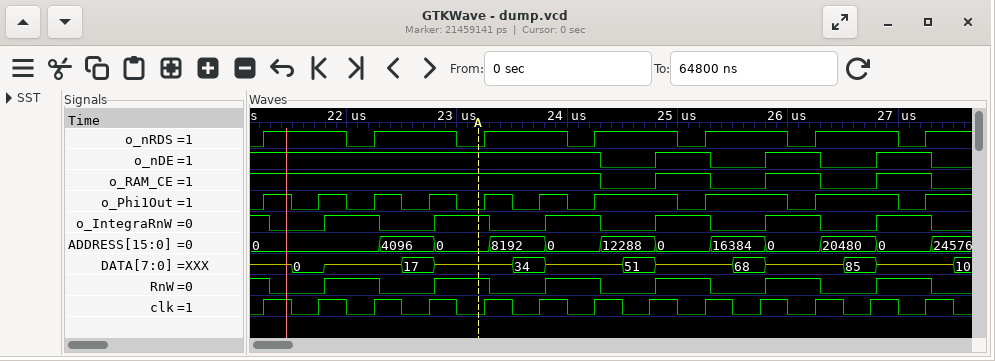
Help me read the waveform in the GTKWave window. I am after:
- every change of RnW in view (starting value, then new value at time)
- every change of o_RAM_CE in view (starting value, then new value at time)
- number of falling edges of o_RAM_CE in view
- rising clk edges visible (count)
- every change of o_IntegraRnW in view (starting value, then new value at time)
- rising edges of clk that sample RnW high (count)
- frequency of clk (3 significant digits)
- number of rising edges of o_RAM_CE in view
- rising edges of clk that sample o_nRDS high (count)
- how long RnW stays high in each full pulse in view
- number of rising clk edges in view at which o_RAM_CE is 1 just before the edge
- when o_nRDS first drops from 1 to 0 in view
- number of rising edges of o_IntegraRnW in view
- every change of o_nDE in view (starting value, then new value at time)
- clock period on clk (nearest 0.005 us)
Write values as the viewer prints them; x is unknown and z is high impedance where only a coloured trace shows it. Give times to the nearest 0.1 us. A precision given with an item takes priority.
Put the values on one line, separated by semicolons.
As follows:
1, 0 at 21.3 us, 1 at 21.8 us, 0 at 22.3 us, 1 at 22.8 us, 0 at 23.3 us, 1 at 23.8 us, 0 at 24.3 us, 1 at 24.8 us, 0 at 25.3 us, 1 at 25.8 us, 0 at 26.3 us, 1 at 26.8 us, 0 at 27.3 us; 1, 0 at 24.3 us, 1 at 24.8 us, 0 at 25.3 us, 1 at 25.8 us, 0 at 26.3 us, 1 at 26.8 us, 0 at 27.3 us; 4; 13; 1, 0 at 21.3 us, 1 at 21.8 us, 0 at 22.3 us, 1 at 22.8 us, 0 at 23.3 us, 1 at 23.8 us, 0 at 24.3 us, 1 at 24.8 us, 0 at 25.3 us, 1 at 25.8 us, 0 at 26.3 us, 1 at 26.8 us, 0 at 27.3 us; 7; 2.00 MHz; 3; 6; 0.5 us, 0.5 us, 0.5 us, 0.5 us, 0.5 us, 0.5 us; 10; 22 us; 6; 1, 0 at 24.3 us, 1 at 24.8 us, 0 at 25.3 us, 1 at 25.8 us, 0 at 26.3 us, 1 at 26.8 us, 0 at 27.3 us; 0.5 us
